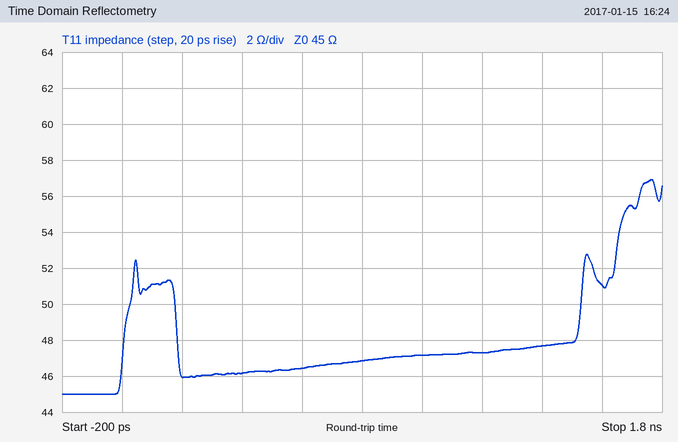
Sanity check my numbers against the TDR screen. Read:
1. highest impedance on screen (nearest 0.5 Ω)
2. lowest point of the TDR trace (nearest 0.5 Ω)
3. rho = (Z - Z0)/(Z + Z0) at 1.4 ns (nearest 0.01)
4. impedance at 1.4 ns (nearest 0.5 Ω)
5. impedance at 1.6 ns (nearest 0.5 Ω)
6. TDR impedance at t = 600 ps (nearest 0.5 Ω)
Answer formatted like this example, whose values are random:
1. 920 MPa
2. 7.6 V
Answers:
1. 57.0 Ω
2. 45.0 Ω
3. +0.03
4. 47.5 Ω
5. 51.0 Ω
6. 46.5 Ω
